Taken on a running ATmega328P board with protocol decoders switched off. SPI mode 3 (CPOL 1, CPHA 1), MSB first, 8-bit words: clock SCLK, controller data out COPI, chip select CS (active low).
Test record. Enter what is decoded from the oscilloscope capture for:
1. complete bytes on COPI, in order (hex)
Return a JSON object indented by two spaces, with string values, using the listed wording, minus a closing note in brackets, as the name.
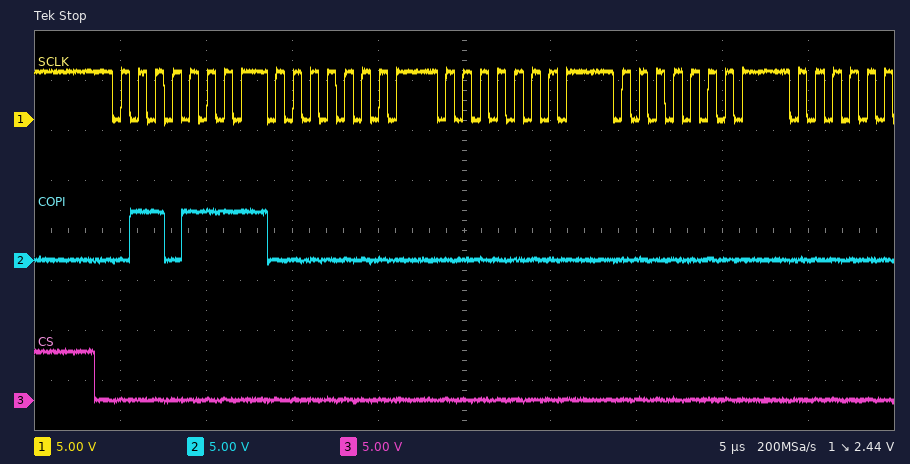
{
  "complete bytes on COPI, in order": "6F 00 00 00"
}
